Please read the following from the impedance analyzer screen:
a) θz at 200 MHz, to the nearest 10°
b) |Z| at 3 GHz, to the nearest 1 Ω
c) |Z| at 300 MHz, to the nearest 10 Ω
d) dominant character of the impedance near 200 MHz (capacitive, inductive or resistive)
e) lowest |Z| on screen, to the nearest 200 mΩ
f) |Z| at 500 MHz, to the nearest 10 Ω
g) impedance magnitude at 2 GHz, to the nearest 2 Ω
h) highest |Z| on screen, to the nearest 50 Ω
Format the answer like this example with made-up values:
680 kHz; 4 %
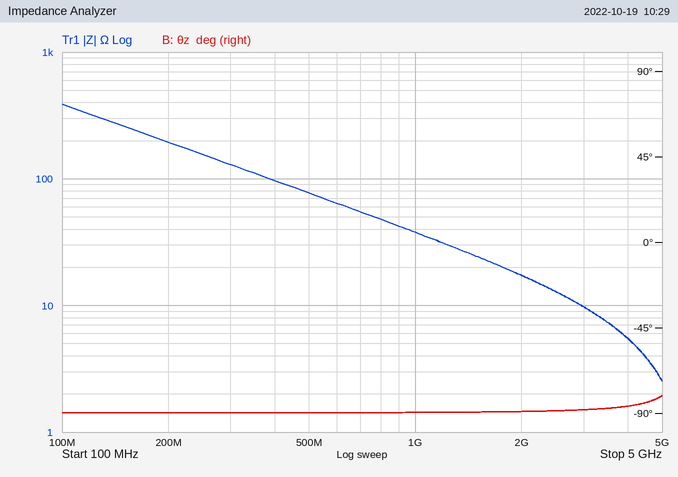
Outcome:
-90°; 10 Ω; 130 Ω; capacitive; 2.6 Ω; 80 Ω; 18 Ω; 400 Ω
